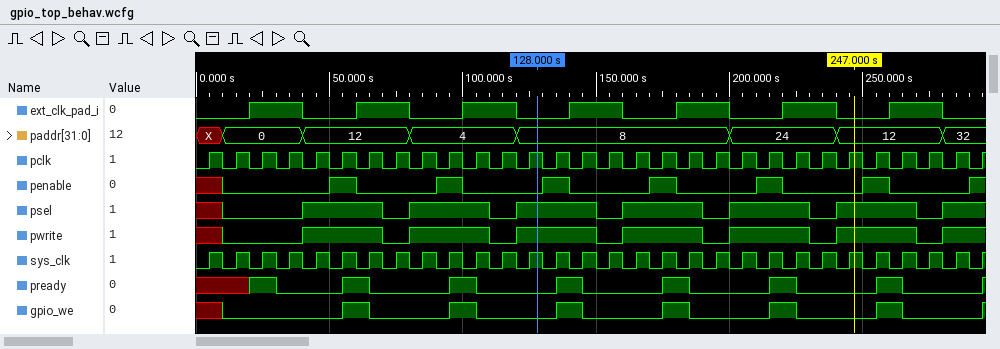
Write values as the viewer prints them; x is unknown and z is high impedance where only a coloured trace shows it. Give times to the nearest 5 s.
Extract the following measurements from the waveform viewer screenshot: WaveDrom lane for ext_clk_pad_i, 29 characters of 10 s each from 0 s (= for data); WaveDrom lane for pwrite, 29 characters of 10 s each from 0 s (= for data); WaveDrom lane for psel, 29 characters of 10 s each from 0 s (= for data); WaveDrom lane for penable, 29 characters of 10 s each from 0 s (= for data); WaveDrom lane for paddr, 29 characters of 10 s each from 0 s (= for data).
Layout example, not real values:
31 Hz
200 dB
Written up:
{name: 'ext_clk_pad_i', wave: '0.1.0.1.0.1.0.1.0.1.0.1.0.1.0'}
{name: 'pwrite', wave: 'x0..1..01..01..01..01..01..01'}
{name: 'psel', wave: 'x0..1..01..01..01..01..01..01'}
{name: 'penable', wave: 'x0...10..10..10..10..10..10..'}
{name: 'paddr', wave: 'x=..=...=...=.......=...=...=', data: '0 12 4 8 24 12 32'}
